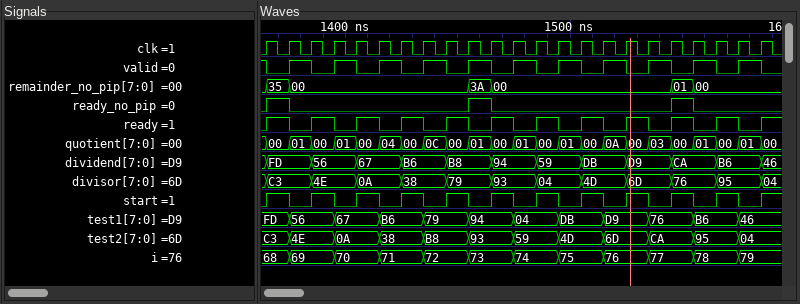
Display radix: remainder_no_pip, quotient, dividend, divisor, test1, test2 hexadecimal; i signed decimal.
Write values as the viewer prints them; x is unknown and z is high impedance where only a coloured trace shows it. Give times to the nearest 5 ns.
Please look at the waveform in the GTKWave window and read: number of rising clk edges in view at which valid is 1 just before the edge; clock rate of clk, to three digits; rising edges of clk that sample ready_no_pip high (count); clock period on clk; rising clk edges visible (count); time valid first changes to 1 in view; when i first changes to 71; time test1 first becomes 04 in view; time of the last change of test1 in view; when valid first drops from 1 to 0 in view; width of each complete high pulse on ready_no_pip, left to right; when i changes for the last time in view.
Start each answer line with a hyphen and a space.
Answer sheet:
- 12
- 100 MHz
- 3
- 10 ns
- 23
- 1375 ns
- 1415 ns
- 1475 ns
- 1575 ns
- 1365 ns
- 10 ns, 10 ns, 10 ns
- 1575 ns
